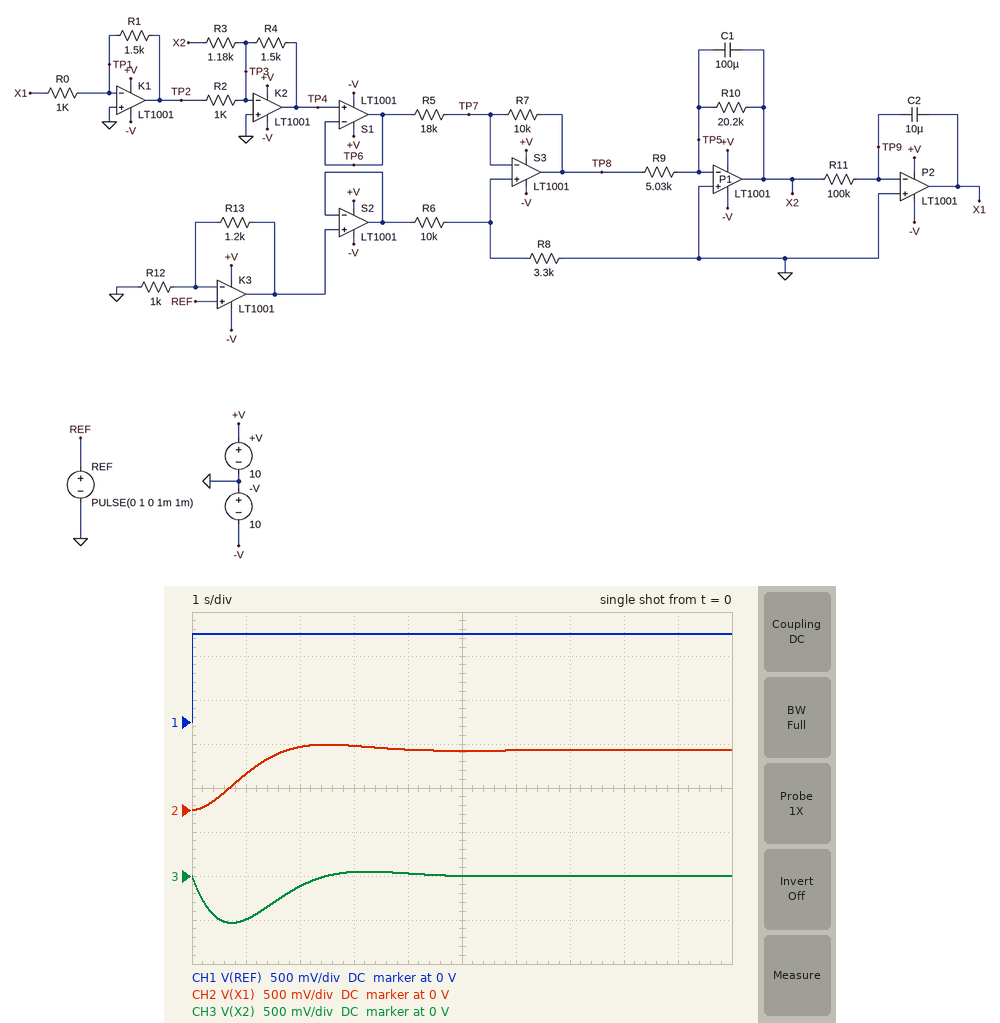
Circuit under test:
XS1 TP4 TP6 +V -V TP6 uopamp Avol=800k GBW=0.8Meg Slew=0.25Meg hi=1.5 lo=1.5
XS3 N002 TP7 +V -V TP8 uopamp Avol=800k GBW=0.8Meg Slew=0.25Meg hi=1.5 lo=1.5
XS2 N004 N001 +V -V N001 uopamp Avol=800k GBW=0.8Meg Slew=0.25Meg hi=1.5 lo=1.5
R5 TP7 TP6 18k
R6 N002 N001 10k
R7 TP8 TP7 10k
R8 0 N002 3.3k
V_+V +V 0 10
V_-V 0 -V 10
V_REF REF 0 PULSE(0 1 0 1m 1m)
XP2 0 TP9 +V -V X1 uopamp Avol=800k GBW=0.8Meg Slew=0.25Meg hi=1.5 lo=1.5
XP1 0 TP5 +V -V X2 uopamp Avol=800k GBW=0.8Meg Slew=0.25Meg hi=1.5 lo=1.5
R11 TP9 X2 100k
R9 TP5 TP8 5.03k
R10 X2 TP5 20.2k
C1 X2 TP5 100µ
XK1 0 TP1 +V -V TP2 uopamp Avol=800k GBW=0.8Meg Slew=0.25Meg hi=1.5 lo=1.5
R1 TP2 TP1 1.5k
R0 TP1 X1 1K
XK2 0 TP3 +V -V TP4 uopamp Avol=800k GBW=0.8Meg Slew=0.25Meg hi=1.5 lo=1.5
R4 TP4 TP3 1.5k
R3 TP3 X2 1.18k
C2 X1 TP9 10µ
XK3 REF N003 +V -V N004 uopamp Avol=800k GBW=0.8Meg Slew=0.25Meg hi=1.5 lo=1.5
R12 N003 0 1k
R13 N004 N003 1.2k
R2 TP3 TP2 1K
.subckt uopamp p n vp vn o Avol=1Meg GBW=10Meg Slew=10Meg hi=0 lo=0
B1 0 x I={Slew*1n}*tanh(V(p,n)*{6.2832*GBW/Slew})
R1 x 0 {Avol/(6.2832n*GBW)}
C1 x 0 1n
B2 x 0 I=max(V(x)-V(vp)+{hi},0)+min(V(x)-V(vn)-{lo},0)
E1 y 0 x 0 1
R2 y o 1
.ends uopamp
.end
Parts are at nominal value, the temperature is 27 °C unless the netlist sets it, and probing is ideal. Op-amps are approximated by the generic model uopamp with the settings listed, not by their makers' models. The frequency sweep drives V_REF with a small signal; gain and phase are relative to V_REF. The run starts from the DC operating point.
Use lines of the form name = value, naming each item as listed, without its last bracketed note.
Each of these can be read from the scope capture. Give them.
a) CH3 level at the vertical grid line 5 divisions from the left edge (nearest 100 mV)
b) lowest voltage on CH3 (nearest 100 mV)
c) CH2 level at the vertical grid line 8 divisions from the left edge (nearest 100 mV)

CH3 level at the vertical grid line 5 divisions from the left edge = 0 V
lowest voltage on CH3 = -500 mV
CH2 level at the vertical grid line 8 divisions from the left edge = 700 mV
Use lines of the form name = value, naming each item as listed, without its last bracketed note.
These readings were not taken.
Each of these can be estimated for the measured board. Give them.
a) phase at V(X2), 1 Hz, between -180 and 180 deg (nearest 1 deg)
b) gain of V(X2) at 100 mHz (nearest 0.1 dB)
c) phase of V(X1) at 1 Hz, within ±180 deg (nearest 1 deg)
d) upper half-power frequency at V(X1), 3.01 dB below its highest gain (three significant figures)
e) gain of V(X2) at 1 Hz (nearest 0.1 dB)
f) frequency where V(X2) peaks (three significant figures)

phase at V(X2), 1 Hz, between -180 and 180 deg = 108 deg
gain of V(X2) at 100 mHz = -7.1 dB
phase of V(X1) at 1 Hz, within ±180 deg = -162 deg
upper half-power frequency at V(X1), 3.01 dB below its highest gain = 279 mHz
gain of V(X2) at 1 Hz = -11.3 dB
frequency where V(X2) peaks = 251 mHz
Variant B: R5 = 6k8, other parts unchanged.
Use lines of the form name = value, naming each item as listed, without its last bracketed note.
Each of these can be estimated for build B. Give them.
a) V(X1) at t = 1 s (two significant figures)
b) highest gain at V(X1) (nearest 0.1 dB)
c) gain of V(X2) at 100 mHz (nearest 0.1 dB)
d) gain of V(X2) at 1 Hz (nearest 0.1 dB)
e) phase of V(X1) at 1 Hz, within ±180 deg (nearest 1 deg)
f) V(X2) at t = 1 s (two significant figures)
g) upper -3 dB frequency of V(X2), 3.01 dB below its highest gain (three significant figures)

V(X1) at t = 1 s = 330 mV
highest gain at V(X1) = -7.8 dB
gain of V(X2) at 100 mHz = -12.0 dB
gain of V(X2) at 1 Hz = -8.0 dB
phase of V(X1) at 1 Hz, within ±180 deg = -141 deg
V(X2) at t = 1 s = -220 mV
upper -3 dB frequency of V(X2), 3.01 dB below its highest gain = 863 mHz
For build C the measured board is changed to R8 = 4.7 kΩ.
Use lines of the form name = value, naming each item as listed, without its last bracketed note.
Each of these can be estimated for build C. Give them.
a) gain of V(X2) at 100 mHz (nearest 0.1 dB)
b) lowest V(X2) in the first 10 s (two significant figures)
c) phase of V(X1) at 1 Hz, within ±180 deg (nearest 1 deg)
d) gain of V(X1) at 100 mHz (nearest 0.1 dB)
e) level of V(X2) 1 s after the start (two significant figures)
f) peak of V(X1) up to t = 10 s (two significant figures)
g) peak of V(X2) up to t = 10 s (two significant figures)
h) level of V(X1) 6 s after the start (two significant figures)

gain of V(X2) at 100 mHz = -4.9 dB
lowest V(X2) in the first 10 s = -690 mV
phase of V(X1) at 1 Hz, within ±180 deg = -162 deg
gain of V(X1) at 100 mHz = -0.9 dB
level of V(X2) 1 s after the start = -640 mV
peak of V(X1) up to t = 10 s = 960 mV
peak of V(X2) up to t = 10 s = 64 mV
level of V(X1) 6 s after the start = 870 mV
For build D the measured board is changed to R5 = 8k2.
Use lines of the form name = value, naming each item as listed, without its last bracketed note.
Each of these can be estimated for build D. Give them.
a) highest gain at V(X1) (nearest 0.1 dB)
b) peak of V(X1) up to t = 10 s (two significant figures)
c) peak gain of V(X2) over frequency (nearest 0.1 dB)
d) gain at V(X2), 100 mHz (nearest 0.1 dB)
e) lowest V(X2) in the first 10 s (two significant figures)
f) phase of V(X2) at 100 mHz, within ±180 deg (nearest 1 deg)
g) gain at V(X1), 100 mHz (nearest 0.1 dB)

highest gain at V(X1) = -7.1 dB
peak of V(X1) up to t = 10 s = 450 mV
peak gain of V(X2) over frequency = -3.4 dB
gain at V(X2), 100 mHz = -11.3 dB
lowest V(X2) in the first 10 s = -450 mV
phase of V(X2) at 100 mHz, within ±180 deg = -114 deg
gain at V(X1), 100 mHz = -7.2 dB
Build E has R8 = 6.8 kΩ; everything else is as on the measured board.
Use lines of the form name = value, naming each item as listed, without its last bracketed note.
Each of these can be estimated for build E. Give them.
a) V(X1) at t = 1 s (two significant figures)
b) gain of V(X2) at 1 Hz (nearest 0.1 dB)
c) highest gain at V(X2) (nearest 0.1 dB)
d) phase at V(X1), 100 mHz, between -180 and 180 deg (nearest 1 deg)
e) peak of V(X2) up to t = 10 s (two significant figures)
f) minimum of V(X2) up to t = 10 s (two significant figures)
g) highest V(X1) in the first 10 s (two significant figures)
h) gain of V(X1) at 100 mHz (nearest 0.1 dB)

V(X1) at t = 1 s = 670 mV
gain of V(X2) at 1 Hz = -7.0 dB
highest gain at V(X2) = 3.2 dB
phase at V(X1), 100 mHz, between -180 and 180 deg = -30 deg
peak of V(X2) up to t = 10 s = 81 mV
minimum of V(X2) up to t = 10 s = -870 mV
highest V(X1) in the first 10 s = 1.2 V
gain of V(X1) at 100 mHz = 1.2 dB
